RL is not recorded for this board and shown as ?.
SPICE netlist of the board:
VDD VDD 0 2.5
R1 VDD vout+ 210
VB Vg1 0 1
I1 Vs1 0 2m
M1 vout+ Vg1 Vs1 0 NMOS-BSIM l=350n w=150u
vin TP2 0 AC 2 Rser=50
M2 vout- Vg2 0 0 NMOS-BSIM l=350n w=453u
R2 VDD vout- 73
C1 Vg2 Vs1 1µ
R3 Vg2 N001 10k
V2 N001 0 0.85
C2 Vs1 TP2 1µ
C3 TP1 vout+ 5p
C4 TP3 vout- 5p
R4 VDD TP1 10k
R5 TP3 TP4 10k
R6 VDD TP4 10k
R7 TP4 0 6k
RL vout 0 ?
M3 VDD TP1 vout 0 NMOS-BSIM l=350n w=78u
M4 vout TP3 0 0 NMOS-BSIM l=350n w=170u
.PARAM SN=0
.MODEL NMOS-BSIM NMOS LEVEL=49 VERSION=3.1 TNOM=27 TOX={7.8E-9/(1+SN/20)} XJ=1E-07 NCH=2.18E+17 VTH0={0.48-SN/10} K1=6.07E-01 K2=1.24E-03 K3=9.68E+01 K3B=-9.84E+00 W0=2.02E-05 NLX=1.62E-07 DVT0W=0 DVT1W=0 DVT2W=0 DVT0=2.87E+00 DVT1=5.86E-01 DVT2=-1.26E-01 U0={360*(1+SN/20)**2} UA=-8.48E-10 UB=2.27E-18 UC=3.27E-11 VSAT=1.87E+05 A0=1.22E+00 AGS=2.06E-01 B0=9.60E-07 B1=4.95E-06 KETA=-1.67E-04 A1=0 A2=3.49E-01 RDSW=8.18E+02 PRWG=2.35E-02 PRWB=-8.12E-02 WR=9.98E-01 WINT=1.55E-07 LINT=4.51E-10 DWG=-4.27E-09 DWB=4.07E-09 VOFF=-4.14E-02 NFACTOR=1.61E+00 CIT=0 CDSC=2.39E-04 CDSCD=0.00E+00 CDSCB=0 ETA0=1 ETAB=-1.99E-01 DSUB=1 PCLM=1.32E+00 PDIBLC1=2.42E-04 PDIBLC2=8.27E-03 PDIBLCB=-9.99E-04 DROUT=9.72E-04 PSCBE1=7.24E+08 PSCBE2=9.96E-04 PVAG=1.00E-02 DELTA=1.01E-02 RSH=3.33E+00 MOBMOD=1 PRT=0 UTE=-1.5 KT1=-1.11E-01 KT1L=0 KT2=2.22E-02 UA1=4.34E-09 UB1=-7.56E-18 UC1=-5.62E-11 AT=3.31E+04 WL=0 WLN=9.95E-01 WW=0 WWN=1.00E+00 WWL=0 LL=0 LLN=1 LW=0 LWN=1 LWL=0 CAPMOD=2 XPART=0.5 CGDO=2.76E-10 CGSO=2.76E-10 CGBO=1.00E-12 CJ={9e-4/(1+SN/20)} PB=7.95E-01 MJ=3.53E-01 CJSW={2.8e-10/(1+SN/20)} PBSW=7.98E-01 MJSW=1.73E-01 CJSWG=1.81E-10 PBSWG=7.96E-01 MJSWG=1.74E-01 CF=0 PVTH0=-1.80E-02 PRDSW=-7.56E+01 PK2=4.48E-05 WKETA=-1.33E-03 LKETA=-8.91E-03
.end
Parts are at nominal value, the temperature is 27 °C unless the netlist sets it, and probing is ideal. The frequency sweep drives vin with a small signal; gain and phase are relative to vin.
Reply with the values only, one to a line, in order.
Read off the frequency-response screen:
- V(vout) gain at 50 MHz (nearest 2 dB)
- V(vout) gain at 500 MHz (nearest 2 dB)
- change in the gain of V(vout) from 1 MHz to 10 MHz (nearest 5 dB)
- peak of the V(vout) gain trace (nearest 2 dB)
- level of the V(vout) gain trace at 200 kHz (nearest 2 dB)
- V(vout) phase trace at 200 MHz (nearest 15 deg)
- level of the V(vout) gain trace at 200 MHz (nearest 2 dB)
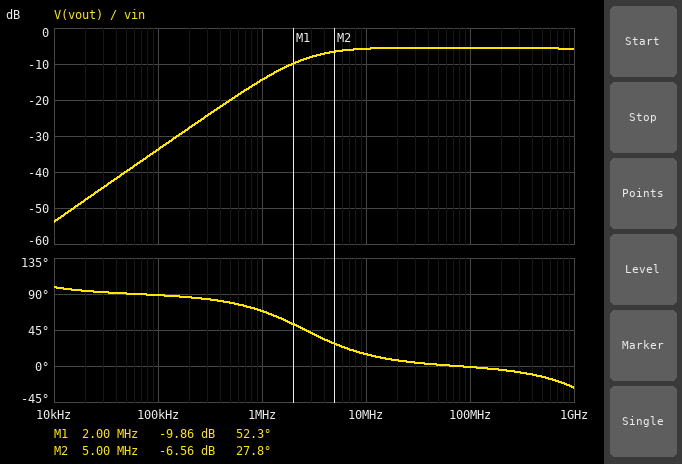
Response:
-6 dB
-6 dB
10 dB
-6 dB
-28 dB
0 deg
-6 dB
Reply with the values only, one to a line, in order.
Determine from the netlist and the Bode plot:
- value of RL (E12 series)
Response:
15 Ω
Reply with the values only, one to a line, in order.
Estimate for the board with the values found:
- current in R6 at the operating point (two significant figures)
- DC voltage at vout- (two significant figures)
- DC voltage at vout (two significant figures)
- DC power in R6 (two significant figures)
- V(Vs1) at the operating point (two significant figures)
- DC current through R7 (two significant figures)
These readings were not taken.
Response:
160 µA
1.9 V
250 mV
240 µW
170 mV
160 µA
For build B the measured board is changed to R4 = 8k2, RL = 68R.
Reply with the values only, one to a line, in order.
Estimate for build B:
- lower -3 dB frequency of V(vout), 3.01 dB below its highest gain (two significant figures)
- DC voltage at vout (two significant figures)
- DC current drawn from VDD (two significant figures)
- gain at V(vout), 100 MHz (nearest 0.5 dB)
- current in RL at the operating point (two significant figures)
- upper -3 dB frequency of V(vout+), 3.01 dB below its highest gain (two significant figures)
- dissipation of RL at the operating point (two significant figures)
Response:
2.9 MHz
610 mV
24 mA
5.0 dB
9.0 mA
3.7 GHz
5.5 mW
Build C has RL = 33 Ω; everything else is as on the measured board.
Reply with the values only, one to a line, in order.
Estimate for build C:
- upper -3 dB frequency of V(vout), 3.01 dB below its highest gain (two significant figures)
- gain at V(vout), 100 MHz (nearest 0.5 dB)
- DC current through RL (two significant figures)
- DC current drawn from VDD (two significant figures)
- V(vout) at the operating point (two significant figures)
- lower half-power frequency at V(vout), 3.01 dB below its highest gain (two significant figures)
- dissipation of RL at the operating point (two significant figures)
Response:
2.9 GHz
1.0 dB
13 mA
27 mA
420 mV
2.6 MHz
5.3 mW
